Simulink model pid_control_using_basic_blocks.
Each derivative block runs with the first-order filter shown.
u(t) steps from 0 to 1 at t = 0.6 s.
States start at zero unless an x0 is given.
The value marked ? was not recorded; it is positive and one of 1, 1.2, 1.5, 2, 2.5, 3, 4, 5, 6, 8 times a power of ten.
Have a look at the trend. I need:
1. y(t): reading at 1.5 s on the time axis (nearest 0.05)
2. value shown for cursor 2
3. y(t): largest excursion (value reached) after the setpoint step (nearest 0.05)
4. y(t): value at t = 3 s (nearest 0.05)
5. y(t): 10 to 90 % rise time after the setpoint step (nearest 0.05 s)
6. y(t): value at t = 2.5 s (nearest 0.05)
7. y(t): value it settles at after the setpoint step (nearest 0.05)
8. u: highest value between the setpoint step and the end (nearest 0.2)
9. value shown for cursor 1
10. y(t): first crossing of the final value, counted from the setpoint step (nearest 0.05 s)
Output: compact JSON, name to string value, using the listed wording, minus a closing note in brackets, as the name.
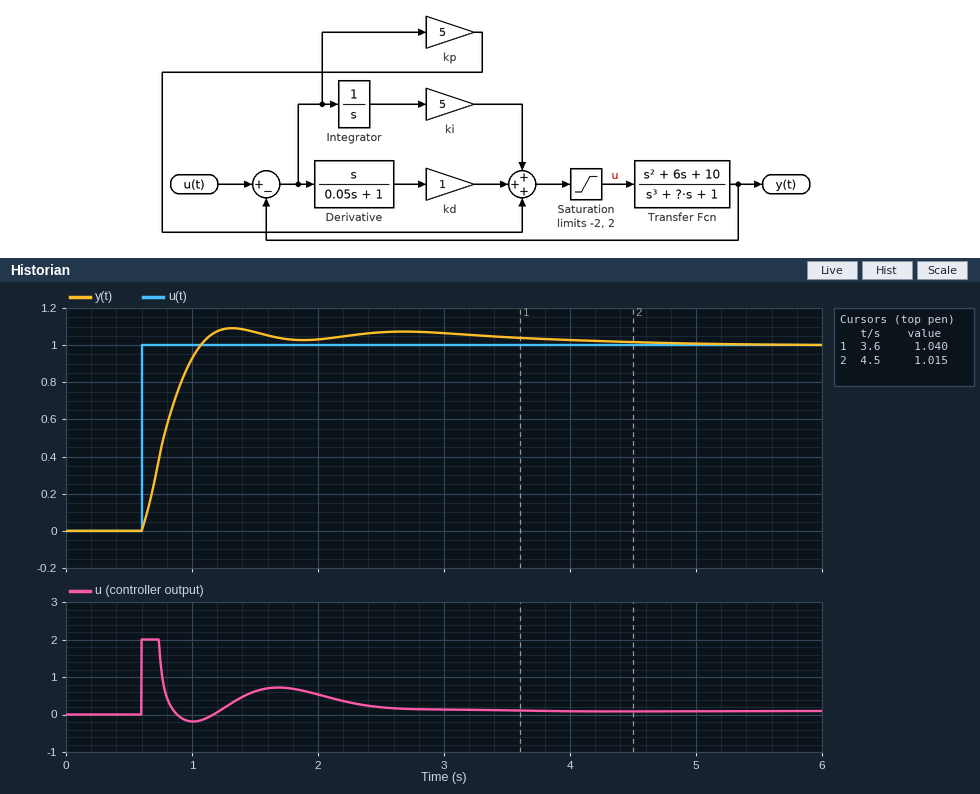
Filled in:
{"y(t): reading at 1.5 s on the time axis": "1.05", "value shown for cursor 2": "1.015", "y(t): largest excursion (value reached) after the setpoint step": "1.10", "y(t): value at t = 3 s": "1.05", "y(t): 10 to 90 % rise time after the setpoint step": "0.35 s", "y(t): value at t = 2.5 s": "1.05", "y(t): value it settles at after the setpoint step": "1.00", "u: highest value between the setpoint step and the end": "2.0", "value shown for cursor 1": "1.040", "y(t): first crossing of the final value, counted from the setpoint step": "0.45 s"}
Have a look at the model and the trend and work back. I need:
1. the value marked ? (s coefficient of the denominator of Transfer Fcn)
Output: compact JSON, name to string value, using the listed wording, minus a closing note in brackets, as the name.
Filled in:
{"the value marked ?": "8"}
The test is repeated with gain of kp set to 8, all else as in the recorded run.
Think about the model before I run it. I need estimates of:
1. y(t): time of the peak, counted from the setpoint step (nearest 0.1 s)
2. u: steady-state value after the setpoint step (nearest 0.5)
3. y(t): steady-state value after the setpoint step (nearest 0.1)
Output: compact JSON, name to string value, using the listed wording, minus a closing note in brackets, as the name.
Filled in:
{"y(t): time of the peak, counted from the setpoint step": "0.6 s", "u: steady-state value after the setpoint step": "0.0", "y(t): steady-state value after the setpoint step": "1.0"}
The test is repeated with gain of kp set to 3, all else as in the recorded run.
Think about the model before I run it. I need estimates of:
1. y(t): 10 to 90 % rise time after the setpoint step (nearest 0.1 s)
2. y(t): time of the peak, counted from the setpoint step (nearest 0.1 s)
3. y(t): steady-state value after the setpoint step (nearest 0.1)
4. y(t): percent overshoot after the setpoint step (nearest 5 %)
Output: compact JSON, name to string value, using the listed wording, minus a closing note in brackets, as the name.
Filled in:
{"y(t): 10 to 90 % rise time after the setpoint step": "0.4 s", "y(t): time of the peak, counted from the setpoint step": "0.9 s", "y(t): steady-state value after the setpoint step": "1.0", "y(t): percent overshoot after the setpoint step": "10 %"}
